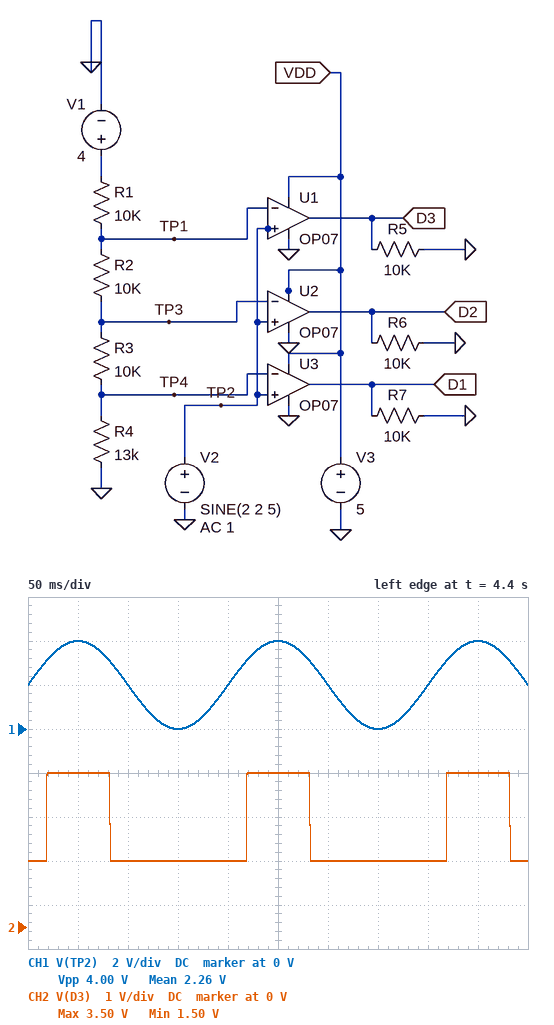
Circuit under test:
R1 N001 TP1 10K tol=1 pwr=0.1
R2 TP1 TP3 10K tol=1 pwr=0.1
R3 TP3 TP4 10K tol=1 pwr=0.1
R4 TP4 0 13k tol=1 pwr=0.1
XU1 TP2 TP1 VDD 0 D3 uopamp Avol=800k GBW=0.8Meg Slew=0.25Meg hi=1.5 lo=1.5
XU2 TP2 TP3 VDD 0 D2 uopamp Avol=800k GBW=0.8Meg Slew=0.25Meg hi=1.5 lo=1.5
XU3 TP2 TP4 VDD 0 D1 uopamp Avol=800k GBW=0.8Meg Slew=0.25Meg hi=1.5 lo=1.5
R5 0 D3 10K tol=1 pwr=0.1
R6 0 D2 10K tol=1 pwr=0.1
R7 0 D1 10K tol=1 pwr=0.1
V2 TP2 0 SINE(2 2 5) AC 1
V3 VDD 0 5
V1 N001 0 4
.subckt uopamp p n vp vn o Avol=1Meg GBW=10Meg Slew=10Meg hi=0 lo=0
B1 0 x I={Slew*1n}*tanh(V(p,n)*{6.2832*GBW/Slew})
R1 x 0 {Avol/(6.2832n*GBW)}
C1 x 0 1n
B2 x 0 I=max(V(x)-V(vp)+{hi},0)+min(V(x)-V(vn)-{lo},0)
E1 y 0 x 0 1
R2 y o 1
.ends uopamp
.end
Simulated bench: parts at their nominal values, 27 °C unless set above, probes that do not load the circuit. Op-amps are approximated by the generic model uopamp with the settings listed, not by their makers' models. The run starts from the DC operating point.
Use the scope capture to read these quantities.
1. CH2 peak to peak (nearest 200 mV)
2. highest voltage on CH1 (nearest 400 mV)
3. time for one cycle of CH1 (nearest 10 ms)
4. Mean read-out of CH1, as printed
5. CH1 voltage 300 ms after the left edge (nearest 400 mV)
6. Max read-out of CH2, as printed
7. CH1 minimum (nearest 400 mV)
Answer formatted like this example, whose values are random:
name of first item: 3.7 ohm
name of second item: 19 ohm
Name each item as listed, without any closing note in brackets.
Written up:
CH2 peak to peak: 2.0 V
highest voltage on CH1: 4.0 V
time for one cycle of CH1: 200 ms
Mean read-out of CH1, as printed: 2.26 V
CH1 voltage 300 ms after the left edge: 2.0 V
Max read-out of CH2, as printed: 3.50 V
CH1 minimum: 0 V
